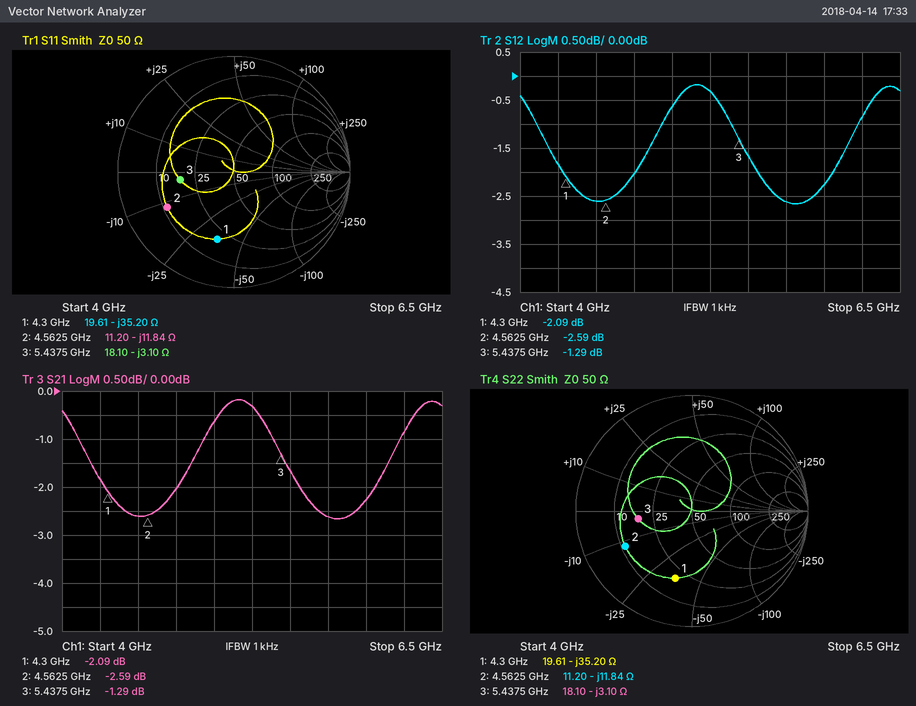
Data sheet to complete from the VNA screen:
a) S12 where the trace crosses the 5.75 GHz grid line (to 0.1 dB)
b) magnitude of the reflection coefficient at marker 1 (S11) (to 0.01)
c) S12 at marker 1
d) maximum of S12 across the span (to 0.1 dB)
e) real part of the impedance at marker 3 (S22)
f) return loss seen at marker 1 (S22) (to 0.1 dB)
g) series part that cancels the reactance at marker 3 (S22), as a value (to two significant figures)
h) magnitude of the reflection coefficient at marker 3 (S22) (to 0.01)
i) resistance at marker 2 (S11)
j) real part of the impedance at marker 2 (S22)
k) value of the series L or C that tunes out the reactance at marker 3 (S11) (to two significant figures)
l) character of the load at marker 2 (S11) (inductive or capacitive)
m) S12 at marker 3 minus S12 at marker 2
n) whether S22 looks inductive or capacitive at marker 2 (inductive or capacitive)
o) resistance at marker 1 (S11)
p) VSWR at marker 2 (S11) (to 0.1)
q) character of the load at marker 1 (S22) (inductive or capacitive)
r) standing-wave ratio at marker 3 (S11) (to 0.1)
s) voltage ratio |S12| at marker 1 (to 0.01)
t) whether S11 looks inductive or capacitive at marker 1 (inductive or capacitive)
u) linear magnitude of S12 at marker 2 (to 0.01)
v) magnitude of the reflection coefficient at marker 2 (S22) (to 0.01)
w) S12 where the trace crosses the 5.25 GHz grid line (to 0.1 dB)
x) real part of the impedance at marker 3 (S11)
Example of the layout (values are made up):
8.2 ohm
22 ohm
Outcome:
-2.6 dB
0.60
-2.09 dB
-0.2 dB
18.10 Ω
4.5 dB
91 pH
0.47
11.20 Ω
11.20 Ω
91 pH
capacitive
1.30 dB
capacitive
19.61 Ω
4.7
capacitive
2.8
0.79
capacitive
0.74
0.65
-0.3 dB
18.10 Ω
